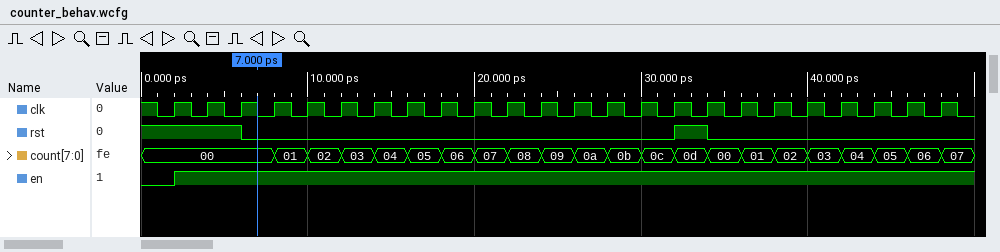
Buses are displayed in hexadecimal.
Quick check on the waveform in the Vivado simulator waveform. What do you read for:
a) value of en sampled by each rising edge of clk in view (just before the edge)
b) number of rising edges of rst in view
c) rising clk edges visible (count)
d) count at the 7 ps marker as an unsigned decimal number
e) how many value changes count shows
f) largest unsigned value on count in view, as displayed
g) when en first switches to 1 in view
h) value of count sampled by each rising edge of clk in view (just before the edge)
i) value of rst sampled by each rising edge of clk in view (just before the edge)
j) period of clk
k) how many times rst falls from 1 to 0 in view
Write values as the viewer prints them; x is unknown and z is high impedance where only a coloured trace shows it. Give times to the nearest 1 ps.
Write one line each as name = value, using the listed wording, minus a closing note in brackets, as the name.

value of en sampled by each rising edge of clk in view = 0 1 1 1 1 1 1 1 1 1 1 1 1 1 1 1 1 1 1 1 1 1 1 1
number of rising edges of rst in view = 1
rising clk edges visible = 24
count at the 7 ps marker as an unsigned decimal number = 0
how many value changes count shows = 21
largest unsigned value on count in view, as displayed = 0d
when en first switches to 1 in view = 2 ps
value of count sampled by each rising edge of clk in view = 00, 00, 00, 00, 01, 02, 03, 04, 05, 06, 07, 08, 09, 0a, 0b, 0c, 0d, 00, 01, 02, 03, 04, 05, 06
value of rst sampled by each rising edge of clk in view = 1 1 1 0 0 0 0 0 0 0 0 0 0 0 0 0 1 0 0 0 0 0 0 0
period of clk = 2 ps
how many times rst falls from 1 to 0 in view = 2
